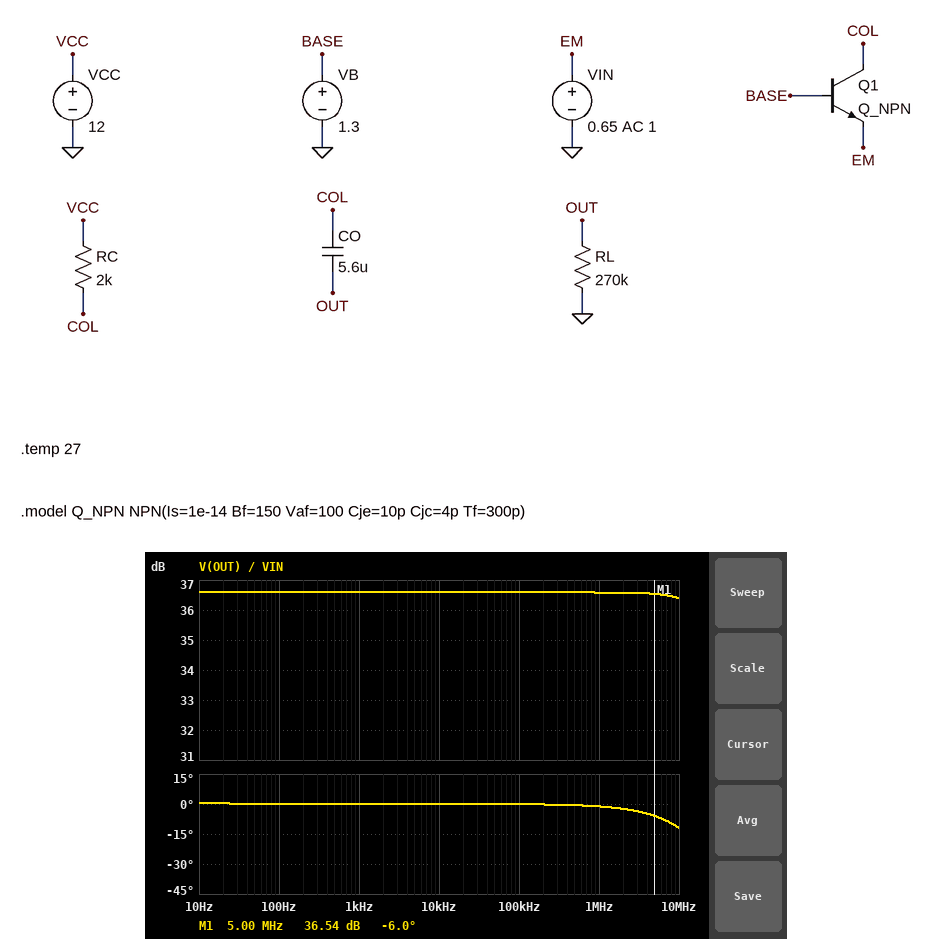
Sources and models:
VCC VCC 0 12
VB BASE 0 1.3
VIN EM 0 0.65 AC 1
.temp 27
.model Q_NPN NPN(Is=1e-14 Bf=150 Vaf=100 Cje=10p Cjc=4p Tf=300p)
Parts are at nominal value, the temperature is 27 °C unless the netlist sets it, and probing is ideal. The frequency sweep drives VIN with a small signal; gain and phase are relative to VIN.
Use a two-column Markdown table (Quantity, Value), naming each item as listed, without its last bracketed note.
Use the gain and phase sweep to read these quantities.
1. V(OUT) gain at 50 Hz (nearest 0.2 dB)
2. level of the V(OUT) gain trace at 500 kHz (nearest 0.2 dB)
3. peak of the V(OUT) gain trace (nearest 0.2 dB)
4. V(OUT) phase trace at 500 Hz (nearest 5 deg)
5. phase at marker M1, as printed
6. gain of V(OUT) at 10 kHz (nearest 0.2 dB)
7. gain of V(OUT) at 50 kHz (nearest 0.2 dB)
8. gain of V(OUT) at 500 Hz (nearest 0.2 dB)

| Quantity | Value |
|---|---|
| V(OUT) gain at 50 Hz | 36.6 dB |
| level of the V(OUT) gain trace at 500 kHz | 36.6 dB |
| peak of the V(OUT) gain trace | 36.6 dB |
| V(OUT) phase trace at 500 Hz | 0 deg |
| phase at marker M1, as printed | -6.0 deg |
| gain of V(OUT) at 10 kHz | 36.6 dB |
| gain of V(OUT) at 50 kHz | 36.6 dB |
| gain of V(OUT) at 500 Hz | 36.6 dB |
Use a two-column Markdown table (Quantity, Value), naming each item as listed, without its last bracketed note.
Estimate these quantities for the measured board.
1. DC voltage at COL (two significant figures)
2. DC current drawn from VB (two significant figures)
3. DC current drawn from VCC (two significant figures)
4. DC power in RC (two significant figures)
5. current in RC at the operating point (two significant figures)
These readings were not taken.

| Quantity | Value |
|---|---|
| DC voltage at COL | 10 V |
| DC current drawn from VB | 5.5 µA |
| DC current drawn from VCC | 890 µA |
| DC power in RC | 1.6 mW |
| current in RC at the operating point | 890 µA |
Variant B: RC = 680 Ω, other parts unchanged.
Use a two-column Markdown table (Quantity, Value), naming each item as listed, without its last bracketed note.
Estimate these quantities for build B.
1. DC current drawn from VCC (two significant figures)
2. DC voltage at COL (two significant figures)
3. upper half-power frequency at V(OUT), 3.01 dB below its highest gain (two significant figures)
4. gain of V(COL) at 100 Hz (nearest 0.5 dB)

| Quantity | Value |
|---|---|
| DC current drawn from VCC | 900 µA |
| DC voltage at COL | 11 V |
| upper half-power frequency at V(OUT), 3.01 dB below its highest gain | 140 MHz |
| gain of V(COL) at 100 Hz | 27.5 dB |
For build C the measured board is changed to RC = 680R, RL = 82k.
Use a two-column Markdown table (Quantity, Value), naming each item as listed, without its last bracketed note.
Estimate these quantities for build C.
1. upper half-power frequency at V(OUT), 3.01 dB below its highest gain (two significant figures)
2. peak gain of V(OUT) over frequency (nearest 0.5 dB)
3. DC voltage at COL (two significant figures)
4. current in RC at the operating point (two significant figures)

| Quantity | Value |
|---|---|
| upper half-power frequency at V(OUT), 3.01 dB below its highest gain | 140 MHz |
| peak gain of V(OUT) over frequency | 27.5 dB |
| DC voltage at COL | 11 V |
| current in RC at the operating point | 900 µA |
